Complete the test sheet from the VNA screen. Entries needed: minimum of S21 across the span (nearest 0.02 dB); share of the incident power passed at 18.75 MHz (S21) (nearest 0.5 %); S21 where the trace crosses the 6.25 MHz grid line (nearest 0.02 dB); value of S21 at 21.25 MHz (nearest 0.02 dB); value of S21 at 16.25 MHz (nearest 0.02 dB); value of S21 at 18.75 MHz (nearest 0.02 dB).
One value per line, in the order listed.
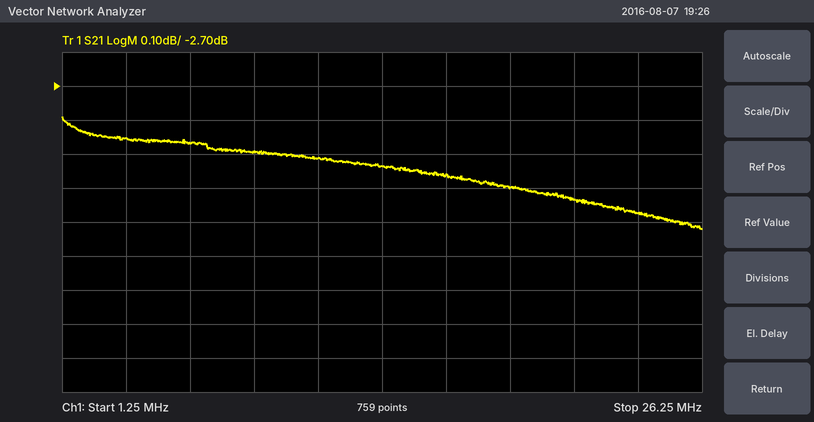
-3.12 dB
50.0 %
-2.86 dB
-3.04 dB
-2.96 dB
-3.00 dB
